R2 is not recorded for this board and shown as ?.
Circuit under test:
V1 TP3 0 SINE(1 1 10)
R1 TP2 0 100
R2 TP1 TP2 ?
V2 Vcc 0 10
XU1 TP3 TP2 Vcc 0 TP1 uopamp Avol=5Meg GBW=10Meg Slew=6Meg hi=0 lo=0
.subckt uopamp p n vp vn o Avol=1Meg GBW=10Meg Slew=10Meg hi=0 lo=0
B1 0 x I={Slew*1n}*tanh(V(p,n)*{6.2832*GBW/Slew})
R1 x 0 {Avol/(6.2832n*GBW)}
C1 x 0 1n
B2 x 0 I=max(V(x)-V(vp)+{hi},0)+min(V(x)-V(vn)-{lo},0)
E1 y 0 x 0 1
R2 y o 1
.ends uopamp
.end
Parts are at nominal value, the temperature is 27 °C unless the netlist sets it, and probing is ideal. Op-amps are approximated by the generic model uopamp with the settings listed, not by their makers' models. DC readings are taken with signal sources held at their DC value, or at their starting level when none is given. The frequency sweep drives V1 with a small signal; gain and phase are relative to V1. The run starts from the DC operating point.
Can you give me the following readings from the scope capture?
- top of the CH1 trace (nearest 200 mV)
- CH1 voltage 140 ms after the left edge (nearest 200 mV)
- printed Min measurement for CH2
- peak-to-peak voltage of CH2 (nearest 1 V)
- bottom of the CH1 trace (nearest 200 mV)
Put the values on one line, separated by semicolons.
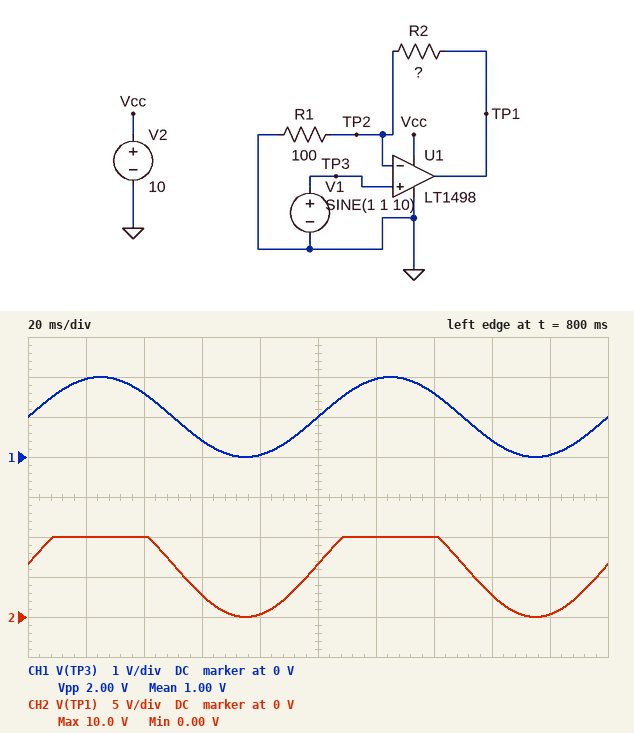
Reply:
2.0 V; 1.6 V; 0.00 V; 10 V; 0 V
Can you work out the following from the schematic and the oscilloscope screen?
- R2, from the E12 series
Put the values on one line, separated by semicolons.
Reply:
560 Ω
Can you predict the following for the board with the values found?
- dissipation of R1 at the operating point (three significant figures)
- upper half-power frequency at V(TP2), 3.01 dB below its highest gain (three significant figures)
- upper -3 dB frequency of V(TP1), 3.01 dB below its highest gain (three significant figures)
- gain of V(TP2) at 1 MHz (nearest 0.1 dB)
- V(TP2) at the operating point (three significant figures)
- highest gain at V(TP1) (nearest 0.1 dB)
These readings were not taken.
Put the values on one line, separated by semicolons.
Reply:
10.0 mW; 1.51 MHz; 1.51 MHz; -1.6 dB; 1.00 V; 16.4 dB
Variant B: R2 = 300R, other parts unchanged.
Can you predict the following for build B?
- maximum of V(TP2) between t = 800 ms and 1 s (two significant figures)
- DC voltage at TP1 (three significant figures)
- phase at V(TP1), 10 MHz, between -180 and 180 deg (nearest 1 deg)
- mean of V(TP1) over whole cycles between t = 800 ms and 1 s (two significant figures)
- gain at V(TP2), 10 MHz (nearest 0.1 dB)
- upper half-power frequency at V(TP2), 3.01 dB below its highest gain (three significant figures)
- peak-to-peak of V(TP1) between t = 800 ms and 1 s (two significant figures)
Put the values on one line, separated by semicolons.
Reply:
2.0 V; 4.00 V; -76 deg; 4.0 V; -12.3 dB; 2.49 MHz; 8.0 V
